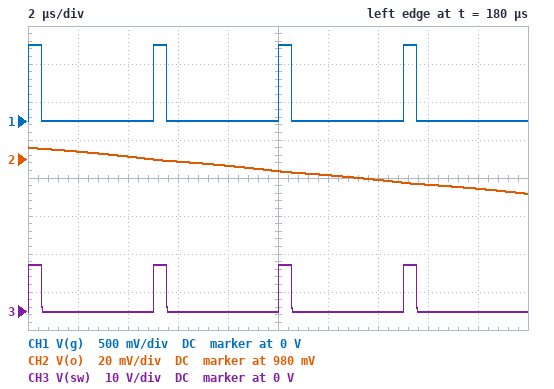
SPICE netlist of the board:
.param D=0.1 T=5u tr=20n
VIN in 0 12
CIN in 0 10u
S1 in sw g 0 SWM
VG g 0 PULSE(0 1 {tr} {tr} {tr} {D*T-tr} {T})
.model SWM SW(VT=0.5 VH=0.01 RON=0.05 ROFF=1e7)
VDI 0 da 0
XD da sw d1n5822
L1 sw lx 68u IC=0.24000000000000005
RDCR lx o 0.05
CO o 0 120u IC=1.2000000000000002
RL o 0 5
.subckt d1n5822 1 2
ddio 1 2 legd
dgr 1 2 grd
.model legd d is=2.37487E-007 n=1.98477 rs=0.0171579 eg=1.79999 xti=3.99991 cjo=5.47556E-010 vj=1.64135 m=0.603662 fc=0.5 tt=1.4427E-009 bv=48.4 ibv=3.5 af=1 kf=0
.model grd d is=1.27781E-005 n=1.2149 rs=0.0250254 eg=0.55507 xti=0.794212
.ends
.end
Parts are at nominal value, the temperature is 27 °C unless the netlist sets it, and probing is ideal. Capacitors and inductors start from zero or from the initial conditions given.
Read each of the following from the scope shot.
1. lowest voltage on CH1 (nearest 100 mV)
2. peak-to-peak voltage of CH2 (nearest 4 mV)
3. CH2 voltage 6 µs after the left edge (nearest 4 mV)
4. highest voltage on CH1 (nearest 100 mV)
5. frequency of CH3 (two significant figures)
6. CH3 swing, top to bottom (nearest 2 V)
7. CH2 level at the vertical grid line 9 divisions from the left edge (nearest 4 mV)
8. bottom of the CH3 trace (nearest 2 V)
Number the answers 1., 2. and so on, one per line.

1. 0 V
2. 24 mV
3. 980 mV
4. 1.0 V
5. 200 kHz
6. 12 V
7. 964 mV
8. 0 V
